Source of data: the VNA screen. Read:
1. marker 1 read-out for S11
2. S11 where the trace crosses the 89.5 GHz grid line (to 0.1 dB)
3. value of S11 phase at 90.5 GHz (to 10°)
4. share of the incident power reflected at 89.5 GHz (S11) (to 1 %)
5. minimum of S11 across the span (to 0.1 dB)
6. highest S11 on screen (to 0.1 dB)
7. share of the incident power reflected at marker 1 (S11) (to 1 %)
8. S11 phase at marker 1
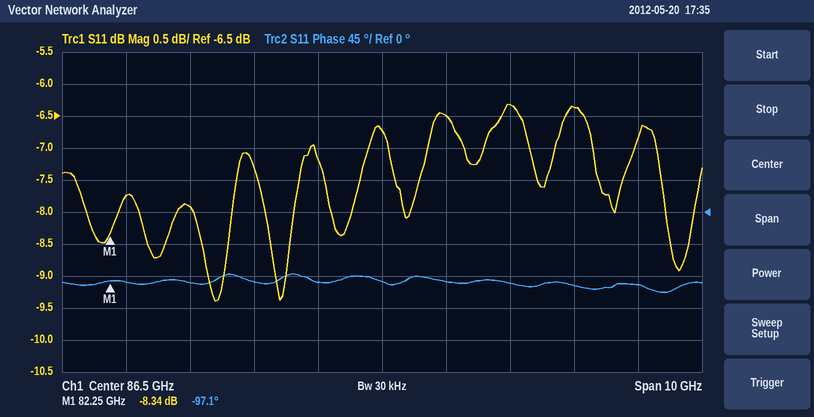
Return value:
-8.34 dB
-6.4 dB
-100°
23 %
-9.4 dB
-6.3 dB
15 %
-97.1°
